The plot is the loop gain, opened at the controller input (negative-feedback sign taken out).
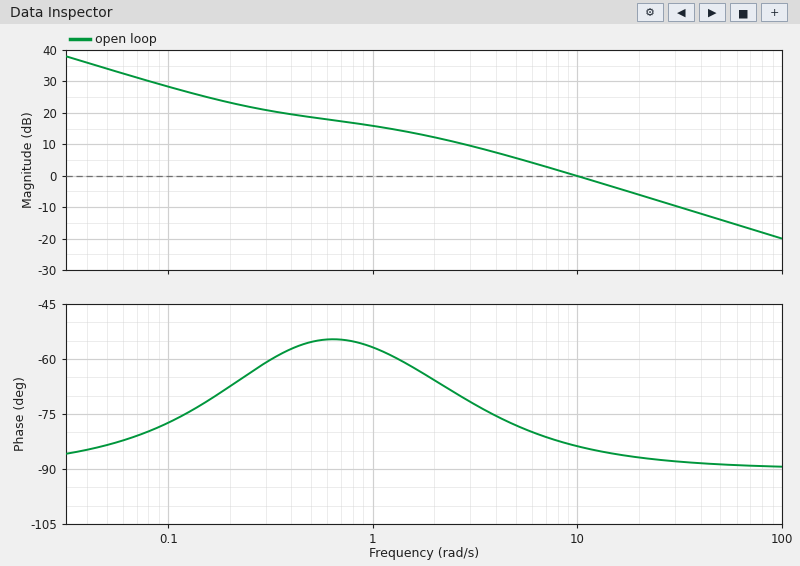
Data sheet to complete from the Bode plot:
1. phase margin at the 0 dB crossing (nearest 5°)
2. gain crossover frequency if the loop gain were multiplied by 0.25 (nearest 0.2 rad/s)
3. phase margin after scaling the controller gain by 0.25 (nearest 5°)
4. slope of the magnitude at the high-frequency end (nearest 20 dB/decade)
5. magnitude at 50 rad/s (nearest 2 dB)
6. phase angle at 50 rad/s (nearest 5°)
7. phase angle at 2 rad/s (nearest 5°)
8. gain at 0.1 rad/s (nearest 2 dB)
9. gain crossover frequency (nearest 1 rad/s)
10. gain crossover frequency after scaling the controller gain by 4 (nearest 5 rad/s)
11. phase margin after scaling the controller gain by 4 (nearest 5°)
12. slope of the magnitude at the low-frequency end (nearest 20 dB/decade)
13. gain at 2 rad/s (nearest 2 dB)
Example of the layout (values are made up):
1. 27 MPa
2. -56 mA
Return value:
1. 95°
2. 2.0 rad/s
3. 115°
4. -20 dB/decade
5. -14 dB
6. -90°
7. -65°
8. 28 dB
9. 10 rad/s
10. 40 rad/s
11. 90°
12. -20 dB/decade
13. 12 dB
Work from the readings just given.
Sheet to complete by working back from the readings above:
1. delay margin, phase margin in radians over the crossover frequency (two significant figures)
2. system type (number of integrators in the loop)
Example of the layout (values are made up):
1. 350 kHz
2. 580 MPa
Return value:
1. 0.17 s
2. 1
